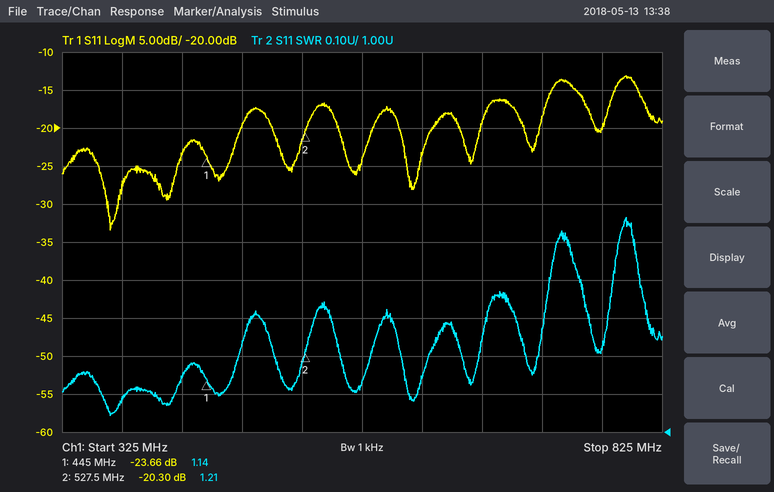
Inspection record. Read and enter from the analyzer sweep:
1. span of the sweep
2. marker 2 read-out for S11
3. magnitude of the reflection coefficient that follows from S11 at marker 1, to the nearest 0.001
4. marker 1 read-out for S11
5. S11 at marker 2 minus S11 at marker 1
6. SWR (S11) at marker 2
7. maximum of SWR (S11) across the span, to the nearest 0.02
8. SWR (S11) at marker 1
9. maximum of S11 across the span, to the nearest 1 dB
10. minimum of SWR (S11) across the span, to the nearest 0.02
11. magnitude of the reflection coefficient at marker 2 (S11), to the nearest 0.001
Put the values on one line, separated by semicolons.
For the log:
500 MHz; -20.30 dB; 0.066; -23.66 dB; 3.36 dB; 1.21; 1.56; 1.14; -13 dB; 1.04; 0.097
